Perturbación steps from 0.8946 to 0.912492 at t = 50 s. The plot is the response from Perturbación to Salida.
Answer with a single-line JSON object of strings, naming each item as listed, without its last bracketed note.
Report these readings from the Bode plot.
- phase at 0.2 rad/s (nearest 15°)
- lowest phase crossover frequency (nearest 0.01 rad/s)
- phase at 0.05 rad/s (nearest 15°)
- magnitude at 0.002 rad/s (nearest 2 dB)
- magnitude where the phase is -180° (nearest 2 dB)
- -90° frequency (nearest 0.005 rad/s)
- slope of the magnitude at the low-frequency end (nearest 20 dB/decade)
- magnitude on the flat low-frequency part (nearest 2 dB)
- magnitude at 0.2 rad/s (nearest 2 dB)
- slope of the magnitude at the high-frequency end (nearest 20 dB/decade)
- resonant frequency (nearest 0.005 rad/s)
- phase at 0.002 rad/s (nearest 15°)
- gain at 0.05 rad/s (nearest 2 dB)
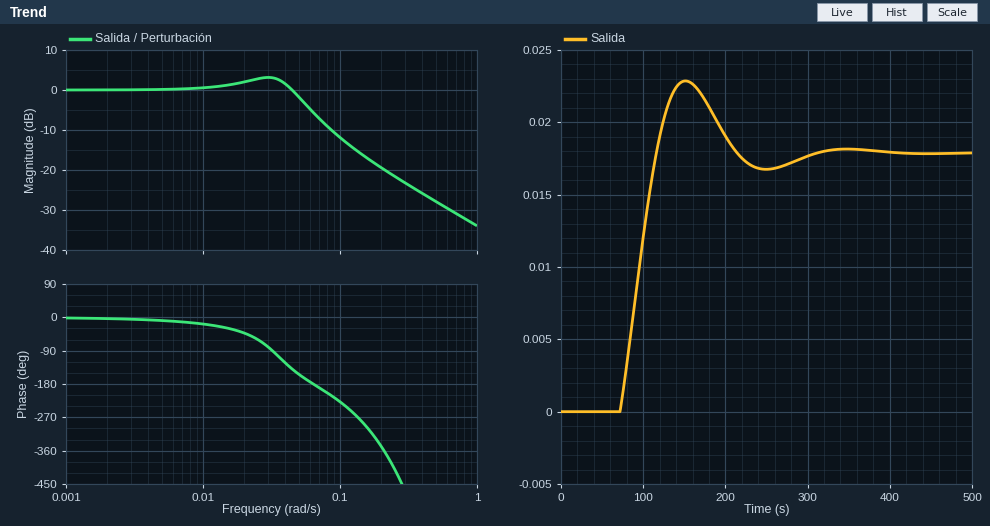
{"phase at 0.2 rad/s": "-345°", "lowest phase crossover frequency": "0.06 rad/s", "phase at 0.05 rad/s": "-150°", "magnitude at 0.002 rad/s": "0 dB", "magnitude where the phase is -180°": "-6 dB", "-90° frequency": "0.030 rad/s", "slope of the magnitude at the low-frequency end": "0 dB/decade", "magnitude on the flat low-frequency part": "0 dB", "magnitude at 0.2 rad/s": "-20 dB", "slope of the magnitude at the high-frequency end": "-20 dB/decade", "resonant frequency": "0.030 rad/s", "phase at 0.002 rad/s": "0°", "gain at 0.05 rad/s": "-2 dB"}
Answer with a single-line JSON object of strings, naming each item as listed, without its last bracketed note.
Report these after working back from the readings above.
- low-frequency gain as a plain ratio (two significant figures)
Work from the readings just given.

{"low-frequency gain as a plain ratio": "1.0"}
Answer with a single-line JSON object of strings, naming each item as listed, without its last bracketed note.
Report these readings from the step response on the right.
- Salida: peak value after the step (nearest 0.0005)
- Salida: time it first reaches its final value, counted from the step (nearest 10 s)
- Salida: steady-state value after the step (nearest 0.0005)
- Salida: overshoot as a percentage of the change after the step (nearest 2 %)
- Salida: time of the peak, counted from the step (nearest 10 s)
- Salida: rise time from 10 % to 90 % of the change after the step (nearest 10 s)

{"Salida: peak value after the step": "0.0230", "Salida: time it first reaches its final value, counted from the step": "70 s", "Salida: steady-state value after the step": "0.0180", "Salida: overshoot as a percentage of the change after the step": "28 %", "Salida: time of the peak, counted from the step": "100 s", "Salida: rise time from 10 % to 90 % of the change after the step": "30 s"}
